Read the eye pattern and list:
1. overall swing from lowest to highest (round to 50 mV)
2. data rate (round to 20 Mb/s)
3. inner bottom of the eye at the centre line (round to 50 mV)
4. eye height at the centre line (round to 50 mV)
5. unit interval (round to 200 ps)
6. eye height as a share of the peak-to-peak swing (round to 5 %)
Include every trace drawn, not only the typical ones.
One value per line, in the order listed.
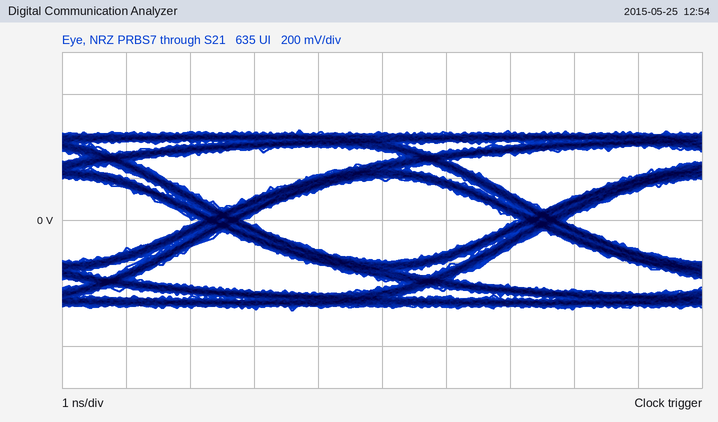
850 mV
200 Mb/s
-200 mV
400 mV
5.0 ns
45 %
